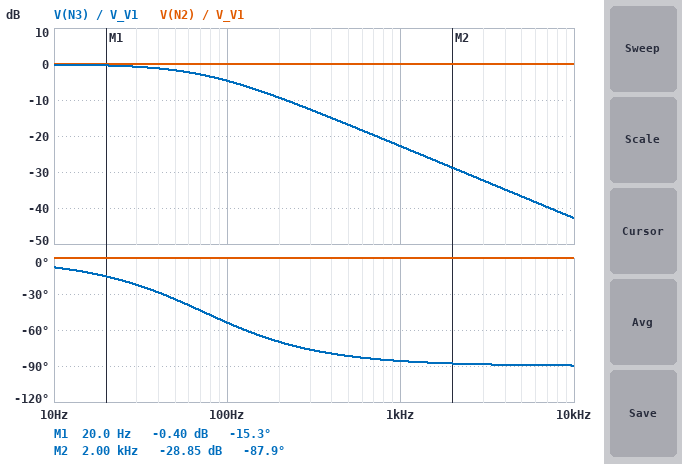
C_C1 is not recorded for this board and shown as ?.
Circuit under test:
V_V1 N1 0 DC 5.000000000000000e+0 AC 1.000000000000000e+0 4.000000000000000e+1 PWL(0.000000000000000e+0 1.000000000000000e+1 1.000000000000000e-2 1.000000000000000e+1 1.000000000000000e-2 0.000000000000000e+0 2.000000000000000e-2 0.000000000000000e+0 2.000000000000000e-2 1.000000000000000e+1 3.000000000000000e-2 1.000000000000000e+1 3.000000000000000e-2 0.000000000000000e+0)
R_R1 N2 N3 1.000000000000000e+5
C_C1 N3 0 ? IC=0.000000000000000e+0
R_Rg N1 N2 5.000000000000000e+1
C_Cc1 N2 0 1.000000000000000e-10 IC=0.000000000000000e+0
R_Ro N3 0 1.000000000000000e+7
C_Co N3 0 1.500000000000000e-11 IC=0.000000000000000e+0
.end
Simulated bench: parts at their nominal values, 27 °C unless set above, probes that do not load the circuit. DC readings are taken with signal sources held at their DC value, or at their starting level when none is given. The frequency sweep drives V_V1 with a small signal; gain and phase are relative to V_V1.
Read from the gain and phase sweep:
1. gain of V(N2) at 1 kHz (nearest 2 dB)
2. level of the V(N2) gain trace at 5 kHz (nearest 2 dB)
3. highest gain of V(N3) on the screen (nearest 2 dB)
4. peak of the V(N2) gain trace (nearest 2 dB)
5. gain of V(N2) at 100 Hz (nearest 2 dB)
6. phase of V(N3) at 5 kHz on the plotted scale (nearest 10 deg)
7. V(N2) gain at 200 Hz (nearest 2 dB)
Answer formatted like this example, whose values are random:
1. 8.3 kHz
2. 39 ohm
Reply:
1. 0 dB
2. 0 dB
3. 0 dB
4. 0 dB
5. 0 dB
6. -90 deg
7. 0 dB
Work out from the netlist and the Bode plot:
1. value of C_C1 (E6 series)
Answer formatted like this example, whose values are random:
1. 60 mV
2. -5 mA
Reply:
1. 22 nF
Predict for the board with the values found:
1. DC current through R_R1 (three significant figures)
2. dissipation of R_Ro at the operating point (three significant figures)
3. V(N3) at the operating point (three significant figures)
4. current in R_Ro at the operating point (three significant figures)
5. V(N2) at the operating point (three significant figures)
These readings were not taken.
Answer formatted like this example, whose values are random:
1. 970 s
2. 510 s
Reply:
1. 495 nA
2. 2.45 µW
3. 4.95 V
4. 495 nA
5. 5.00 V
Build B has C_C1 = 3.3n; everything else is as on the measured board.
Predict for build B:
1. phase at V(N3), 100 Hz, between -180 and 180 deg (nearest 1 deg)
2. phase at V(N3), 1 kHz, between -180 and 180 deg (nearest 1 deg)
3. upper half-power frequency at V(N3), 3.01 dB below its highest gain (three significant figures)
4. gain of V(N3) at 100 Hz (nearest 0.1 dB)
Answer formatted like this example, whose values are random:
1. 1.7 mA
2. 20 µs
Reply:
1. -12 deg
2. -64 deg
3. 485 Hz
4. -0.3 dB
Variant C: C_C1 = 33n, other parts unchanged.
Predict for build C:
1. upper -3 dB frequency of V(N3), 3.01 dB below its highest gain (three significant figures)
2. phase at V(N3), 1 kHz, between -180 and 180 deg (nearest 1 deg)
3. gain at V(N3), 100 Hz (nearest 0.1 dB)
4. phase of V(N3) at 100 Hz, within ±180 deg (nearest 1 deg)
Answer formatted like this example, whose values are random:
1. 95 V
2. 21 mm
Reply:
1. 48.7 Hz
2. -87 deg
3. -7.3 dB
4. -64 deg
